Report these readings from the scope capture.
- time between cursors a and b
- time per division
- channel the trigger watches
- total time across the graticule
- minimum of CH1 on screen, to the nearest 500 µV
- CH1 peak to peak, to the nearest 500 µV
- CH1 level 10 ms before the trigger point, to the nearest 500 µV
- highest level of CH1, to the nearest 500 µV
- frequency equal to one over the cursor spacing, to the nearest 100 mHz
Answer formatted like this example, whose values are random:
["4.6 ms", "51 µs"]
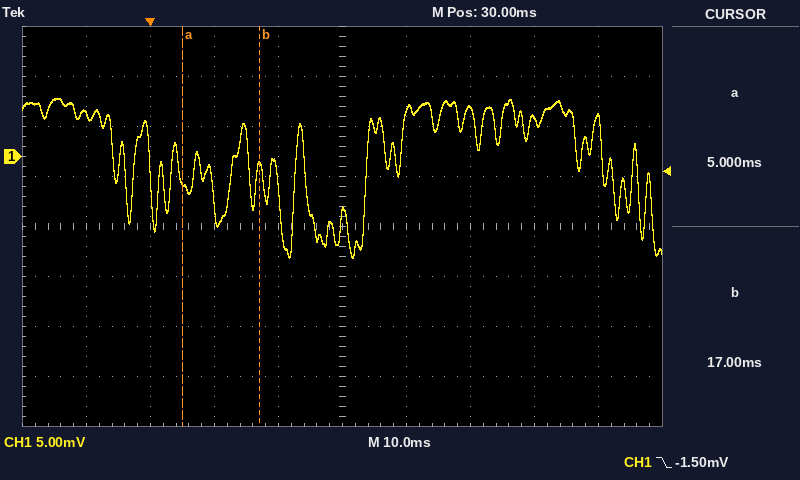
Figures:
["12 ms", "10 ms", "CH1", "100 ms", "-10.0 mV", "16.0 mV", "4.0 mV", "6.0 mV", "83.3 Hz"]
